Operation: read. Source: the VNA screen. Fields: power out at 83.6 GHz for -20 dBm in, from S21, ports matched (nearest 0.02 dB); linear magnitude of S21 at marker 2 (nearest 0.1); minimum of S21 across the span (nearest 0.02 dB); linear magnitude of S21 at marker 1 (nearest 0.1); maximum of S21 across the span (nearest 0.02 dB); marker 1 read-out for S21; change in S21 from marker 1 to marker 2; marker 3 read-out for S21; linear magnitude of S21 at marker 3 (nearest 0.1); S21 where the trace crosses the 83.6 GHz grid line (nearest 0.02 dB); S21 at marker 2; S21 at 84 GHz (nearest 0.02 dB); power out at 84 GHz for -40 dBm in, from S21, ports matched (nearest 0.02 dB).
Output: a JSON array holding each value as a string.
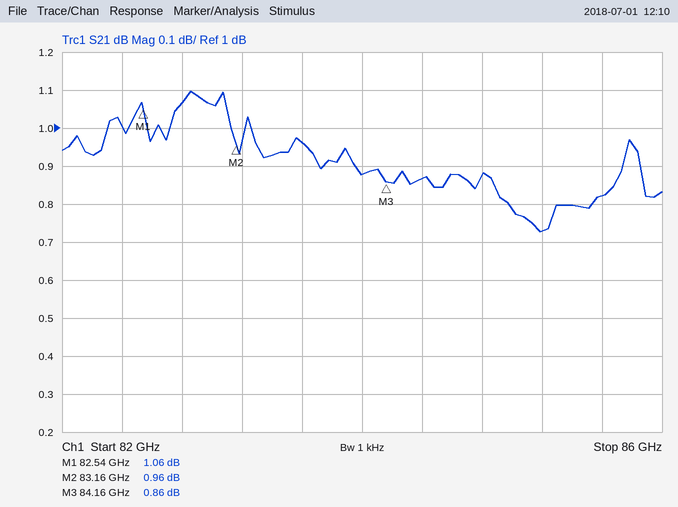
["-19.04 dBm", "1.1", "0.72 dB", "1.1", "1.10 dB", "1.06 dB", "-0.10 dB", "0.86 dB", "1.1", "0.96 dB", "0.96 dB", "0.88 dB", "-39.12 dBm"]
